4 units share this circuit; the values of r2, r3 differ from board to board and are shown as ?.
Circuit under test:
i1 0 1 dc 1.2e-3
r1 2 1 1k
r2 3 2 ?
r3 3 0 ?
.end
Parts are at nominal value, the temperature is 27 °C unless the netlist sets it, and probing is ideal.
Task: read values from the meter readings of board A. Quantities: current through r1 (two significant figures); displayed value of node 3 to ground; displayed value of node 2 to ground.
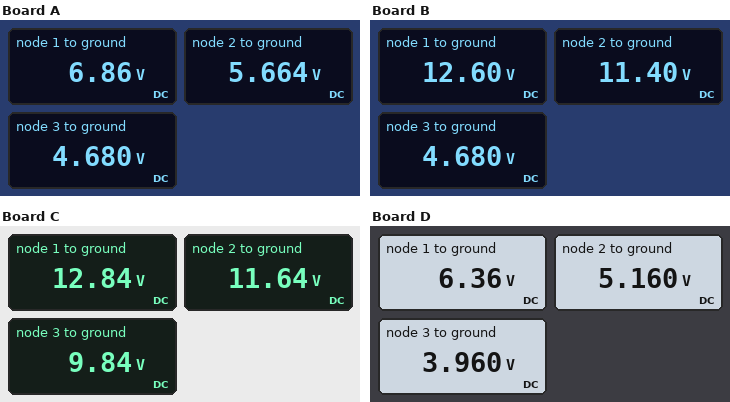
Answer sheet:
1.2 mA
4.680 V
5.664 V
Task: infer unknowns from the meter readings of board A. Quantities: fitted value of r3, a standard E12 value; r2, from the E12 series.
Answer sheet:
3.9 kΩ
820 Ω
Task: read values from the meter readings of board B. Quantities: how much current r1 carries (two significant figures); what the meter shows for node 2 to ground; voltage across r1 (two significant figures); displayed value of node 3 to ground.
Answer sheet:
1.2 mA
11.40 V
1.2 V
4.680 V
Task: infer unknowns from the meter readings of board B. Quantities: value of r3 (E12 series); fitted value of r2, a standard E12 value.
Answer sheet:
3.9 kΩ
5.6 kΩ
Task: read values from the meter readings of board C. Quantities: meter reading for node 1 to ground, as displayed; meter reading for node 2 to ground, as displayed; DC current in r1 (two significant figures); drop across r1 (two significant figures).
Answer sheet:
12.84 V
11.64 V
1.2 mA
1.2 V
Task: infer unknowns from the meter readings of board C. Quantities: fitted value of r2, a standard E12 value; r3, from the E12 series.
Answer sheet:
1.5 kΩ
8.2 kΩ
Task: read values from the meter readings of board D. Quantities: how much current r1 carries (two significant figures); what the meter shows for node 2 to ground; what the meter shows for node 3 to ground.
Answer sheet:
1.2 mA
5.160 V
3.960 V
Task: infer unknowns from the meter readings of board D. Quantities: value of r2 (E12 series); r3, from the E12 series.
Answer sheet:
1 kΩ
3.3 kΩ
